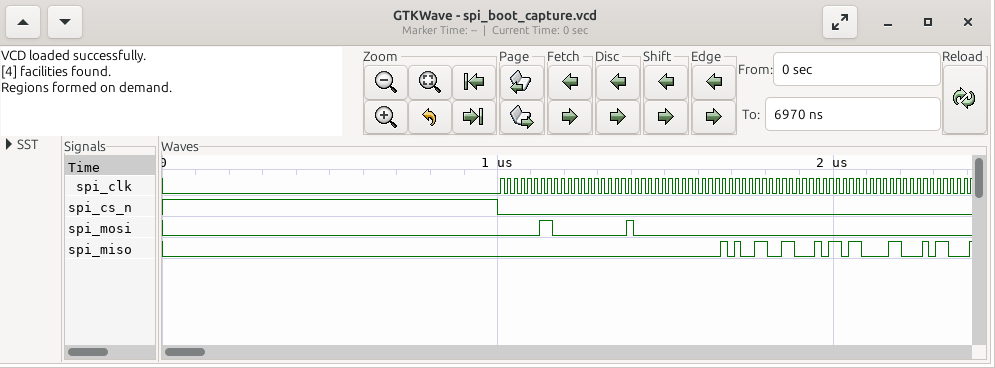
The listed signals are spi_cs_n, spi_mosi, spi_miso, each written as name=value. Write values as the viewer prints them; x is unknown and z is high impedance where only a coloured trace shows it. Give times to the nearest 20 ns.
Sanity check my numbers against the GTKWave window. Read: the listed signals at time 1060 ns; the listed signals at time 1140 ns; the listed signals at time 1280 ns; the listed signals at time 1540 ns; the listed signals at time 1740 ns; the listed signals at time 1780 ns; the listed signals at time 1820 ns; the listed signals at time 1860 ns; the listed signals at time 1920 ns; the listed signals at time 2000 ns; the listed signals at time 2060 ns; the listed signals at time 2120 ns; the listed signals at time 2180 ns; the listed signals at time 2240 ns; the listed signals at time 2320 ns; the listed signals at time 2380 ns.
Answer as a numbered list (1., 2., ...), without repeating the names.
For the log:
1. spi_cs_n=0, spi_mosi=0, spi_miso=0
2. spi_cs_n=0, spi_mosi=1, spi_miso=0
3. spi_cs_n=0, spi_mosi=0, spi_miso=0
4. spi_cs_n=0, spi_mosi=0, spi_miso=0
5. spi_cs_n=0, spi_mosi=0, spi_miso=0
6. spi_cs_n=0, spi_mosi=0, spi_miso=1
7. spi_cs_n=0, spi_mosi=0, spi_miso=0
8. spi_cs_n=0, spi_mosi=0, spi_miso=1
9. spi_cs_n=0, spi_mosi=0, spi_miso=0
10. spi_cs_n=0, spi_mosi=0, spi_miso=1
11. spi_cs_n=0, spi_mosi=0, spi_miso=1
12. spi_cs_n=0, spi_mosi=0, spi_miso=0
13. spi_cs_n=0, spi_mosi=0, spi_miso=1
14. spi_cs_n=0, spi_mosi=0, spi_miso=0
15. spi_cs_n=0, spi_mosi=0, spi_miso=1
16. spi_cs_n=0, spi_mosi=0, spi_miso=0
